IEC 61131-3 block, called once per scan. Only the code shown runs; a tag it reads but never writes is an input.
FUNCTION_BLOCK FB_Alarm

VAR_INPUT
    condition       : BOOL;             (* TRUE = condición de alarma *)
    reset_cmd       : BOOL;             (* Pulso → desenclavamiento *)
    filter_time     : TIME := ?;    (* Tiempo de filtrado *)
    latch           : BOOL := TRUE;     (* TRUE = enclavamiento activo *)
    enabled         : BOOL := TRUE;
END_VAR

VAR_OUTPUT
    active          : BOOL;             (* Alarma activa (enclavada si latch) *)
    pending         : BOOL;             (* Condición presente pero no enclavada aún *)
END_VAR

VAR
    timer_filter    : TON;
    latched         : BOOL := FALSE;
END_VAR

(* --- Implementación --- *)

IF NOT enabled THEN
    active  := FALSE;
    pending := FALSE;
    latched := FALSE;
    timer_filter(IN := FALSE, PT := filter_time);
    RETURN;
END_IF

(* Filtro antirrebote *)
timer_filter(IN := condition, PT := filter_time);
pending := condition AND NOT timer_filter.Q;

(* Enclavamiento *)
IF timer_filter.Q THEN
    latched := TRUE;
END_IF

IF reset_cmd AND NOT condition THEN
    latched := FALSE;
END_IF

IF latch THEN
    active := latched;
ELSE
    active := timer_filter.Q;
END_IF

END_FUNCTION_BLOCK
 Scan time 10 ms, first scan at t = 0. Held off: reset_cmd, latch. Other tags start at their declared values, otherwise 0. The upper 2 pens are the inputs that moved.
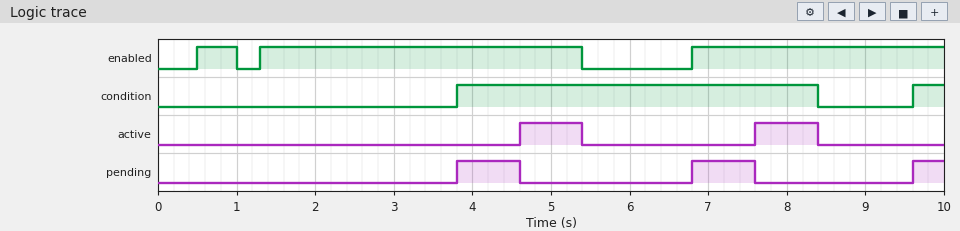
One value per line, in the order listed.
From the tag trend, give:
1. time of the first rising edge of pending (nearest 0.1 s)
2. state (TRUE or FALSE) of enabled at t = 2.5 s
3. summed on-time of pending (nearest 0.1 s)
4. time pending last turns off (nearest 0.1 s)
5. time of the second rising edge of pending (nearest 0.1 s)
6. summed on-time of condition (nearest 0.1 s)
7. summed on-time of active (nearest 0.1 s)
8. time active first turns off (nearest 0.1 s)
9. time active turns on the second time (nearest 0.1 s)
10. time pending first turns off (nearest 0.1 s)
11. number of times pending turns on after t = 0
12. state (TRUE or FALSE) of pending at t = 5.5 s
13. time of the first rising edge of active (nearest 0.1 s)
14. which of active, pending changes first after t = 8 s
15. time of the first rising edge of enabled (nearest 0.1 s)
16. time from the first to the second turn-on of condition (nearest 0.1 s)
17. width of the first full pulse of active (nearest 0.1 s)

3.8 s
TRUE
2.0 s
7.6 s
6.8 s
5.0 s
1.6 s
5.4 s
7.6 s
4.6 s
3
FALSE
4.6 s
active
0.5 s
5.8 s
0.8 s
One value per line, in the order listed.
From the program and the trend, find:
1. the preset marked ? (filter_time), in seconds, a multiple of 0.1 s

0.8 s
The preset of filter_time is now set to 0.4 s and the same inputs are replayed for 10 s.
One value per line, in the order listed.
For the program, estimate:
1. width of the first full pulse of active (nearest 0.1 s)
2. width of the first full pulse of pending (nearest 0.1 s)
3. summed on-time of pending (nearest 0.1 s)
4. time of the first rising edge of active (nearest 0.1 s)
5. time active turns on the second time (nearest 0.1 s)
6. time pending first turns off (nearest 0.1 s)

1.2 s
0.4 s
1.2 s
4.2 s
7.2 s
4.2 s
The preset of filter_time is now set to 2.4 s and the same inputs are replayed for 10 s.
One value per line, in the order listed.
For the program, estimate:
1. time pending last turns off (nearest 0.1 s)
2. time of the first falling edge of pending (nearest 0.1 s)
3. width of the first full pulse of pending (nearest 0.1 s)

8.4 s
5.4 s
1.6 s
